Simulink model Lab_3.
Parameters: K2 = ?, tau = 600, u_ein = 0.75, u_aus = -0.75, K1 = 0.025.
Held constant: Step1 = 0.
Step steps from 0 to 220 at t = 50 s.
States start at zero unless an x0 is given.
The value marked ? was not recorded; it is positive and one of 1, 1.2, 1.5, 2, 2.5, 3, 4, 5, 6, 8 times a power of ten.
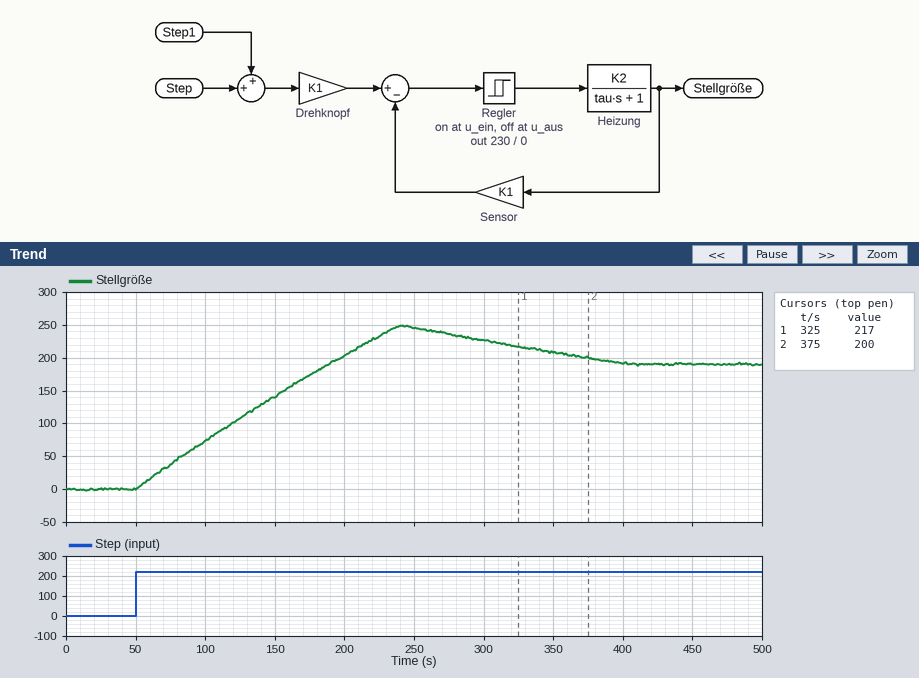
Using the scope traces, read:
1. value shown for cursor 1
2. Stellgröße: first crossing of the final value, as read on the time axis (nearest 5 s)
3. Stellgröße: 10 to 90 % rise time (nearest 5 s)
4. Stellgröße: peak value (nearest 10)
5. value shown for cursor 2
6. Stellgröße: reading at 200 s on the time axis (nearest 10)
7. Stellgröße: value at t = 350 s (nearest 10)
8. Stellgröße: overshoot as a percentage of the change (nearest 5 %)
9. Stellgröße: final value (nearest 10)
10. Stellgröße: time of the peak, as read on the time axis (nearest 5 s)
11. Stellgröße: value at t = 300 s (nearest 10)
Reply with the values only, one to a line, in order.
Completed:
217
190 s
110 s
250
200
200
210
30 %
190
240 s
230
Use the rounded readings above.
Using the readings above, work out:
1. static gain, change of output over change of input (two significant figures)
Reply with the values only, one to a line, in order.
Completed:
0.86
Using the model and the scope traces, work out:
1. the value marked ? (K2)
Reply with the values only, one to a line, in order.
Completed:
4
